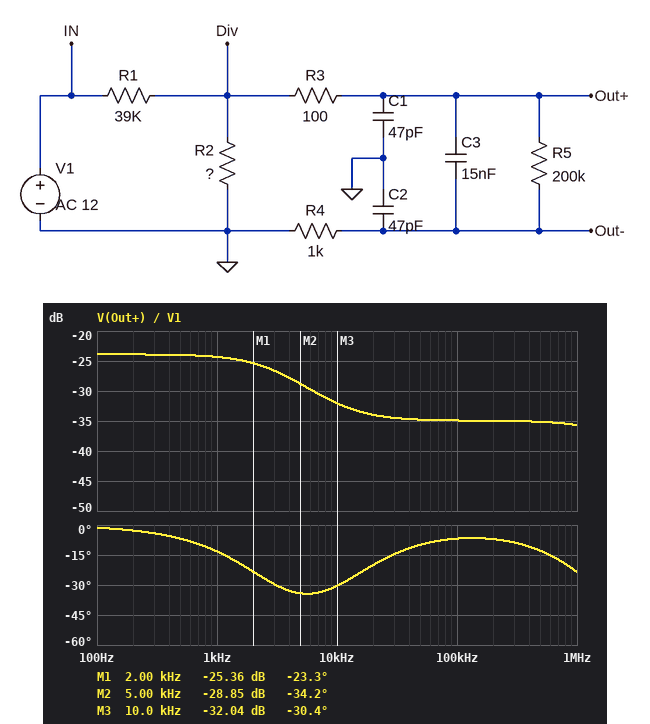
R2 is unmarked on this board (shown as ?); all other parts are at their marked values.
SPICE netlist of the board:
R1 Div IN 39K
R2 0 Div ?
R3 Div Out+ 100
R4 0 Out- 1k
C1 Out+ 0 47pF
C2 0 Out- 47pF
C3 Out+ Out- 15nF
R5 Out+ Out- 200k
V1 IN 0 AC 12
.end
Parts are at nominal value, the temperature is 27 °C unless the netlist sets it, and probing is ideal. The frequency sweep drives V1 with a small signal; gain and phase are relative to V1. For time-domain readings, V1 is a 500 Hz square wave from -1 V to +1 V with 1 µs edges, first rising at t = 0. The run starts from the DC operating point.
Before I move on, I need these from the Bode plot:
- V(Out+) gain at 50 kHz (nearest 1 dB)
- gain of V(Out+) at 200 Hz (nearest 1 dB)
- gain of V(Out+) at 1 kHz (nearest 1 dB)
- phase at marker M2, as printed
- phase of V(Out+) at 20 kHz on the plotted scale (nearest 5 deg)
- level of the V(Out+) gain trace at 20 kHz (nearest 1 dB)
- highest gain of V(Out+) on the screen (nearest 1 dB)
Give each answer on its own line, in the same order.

-35 dB
-24 dB
-24 dB
-34.2 deg
-20 deg
-34 dB
-24 dB
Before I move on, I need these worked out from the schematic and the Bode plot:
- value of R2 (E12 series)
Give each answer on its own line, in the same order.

2.7 kΩ
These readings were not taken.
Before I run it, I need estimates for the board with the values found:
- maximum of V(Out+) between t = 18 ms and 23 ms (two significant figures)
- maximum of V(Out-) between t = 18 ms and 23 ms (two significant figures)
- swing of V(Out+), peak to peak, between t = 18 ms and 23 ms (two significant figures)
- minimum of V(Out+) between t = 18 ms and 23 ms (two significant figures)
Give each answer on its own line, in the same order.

64 mV
35 mV
130 mV
-64 mV
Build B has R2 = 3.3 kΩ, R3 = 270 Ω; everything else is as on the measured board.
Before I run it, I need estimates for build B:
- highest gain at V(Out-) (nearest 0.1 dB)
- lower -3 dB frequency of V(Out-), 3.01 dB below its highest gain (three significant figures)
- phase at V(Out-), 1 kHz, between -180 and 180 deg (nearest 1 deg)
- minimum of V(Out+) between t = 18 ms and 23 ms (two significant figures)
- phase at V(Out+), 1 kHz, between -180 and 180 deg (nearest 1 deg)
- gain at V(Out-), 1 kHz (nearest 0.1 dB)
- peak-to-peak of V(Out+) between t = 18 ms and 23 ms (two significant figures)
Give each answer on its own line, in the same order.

-34.9 dB
2.50 kHz
65 deg
-77 mV
-16 deg
-43.5 dB
150 mV
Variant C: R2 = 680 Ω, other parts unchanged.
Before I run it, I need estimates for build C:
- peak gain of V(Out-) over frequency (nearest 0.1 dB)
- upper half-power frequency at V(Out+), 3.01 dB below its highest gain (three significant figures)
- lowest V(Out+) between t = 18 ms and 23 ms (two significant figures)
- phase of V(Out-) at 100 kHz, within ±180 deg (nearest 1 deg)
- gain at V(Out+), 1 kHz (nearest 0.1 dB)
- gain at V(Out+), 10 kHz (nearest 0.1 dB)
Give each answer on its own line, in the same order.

-40.3 dB
10.2 kHz
-17 mV
2 deg
-35.4 dB
-38.3 dB
